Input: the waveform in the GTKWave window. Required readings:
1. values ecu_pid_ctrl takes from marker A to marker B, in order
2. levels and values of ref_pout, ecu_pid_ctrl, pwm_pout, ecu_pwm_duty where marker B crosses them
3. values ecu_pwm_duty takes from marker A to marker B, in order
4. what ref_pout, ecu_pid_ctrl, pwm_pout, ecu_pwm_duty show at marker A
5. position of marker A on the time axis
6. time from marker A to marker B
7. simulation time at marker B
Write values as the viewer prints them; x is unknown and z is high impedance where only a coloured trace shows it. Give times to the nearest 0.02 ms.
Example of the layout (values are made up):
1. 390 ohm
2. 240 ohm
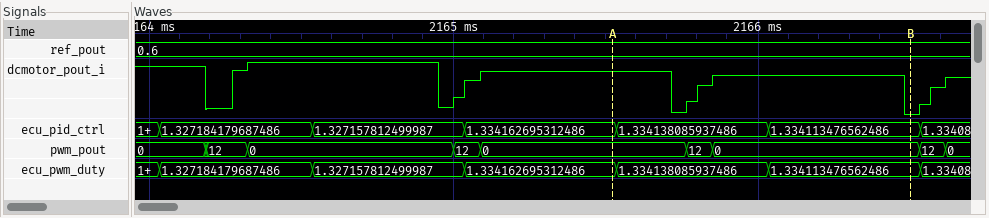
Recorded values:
1. 1.334162695312486, 1.334138085937486, 1.334113476562486
2. ref_pout=0.6, ecu_pid_ctrl=1.334113476562486, pwm_pout=0, ecu_pwm_duty=1.334113476562486
3. 1.334162695312486, 1.334138085937486, 1.334113476562486
4. ref_pout=0.6, ecu_pid_ctrl=1.334162695312486, pwm_pout=0, ecu_pwm_duty=1.334162695312486
5. 2165.52 ms
6. 0.98 ms
7. 2166.5 ms
